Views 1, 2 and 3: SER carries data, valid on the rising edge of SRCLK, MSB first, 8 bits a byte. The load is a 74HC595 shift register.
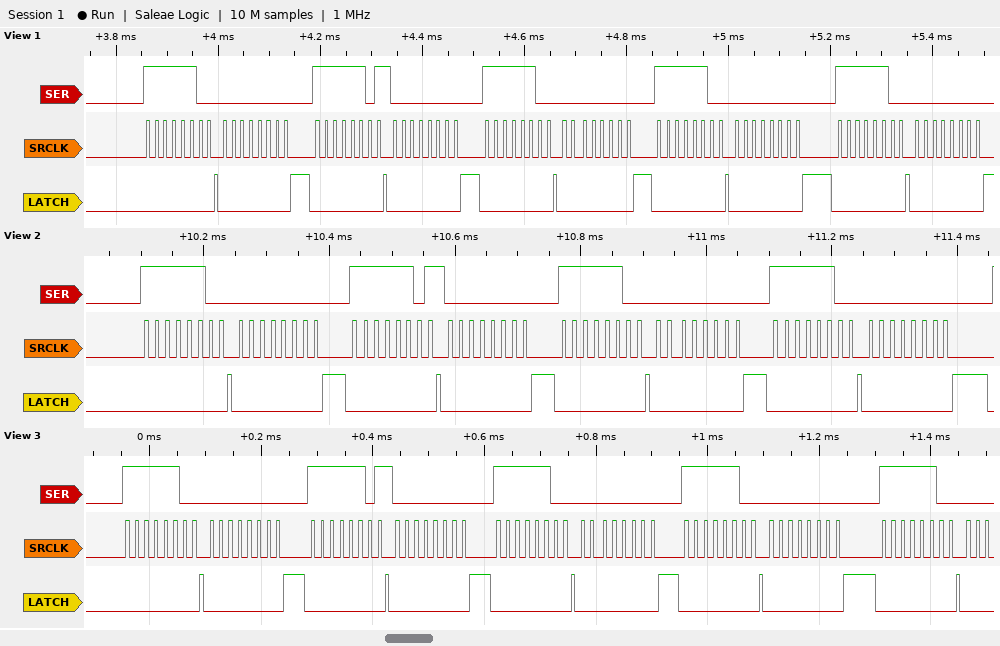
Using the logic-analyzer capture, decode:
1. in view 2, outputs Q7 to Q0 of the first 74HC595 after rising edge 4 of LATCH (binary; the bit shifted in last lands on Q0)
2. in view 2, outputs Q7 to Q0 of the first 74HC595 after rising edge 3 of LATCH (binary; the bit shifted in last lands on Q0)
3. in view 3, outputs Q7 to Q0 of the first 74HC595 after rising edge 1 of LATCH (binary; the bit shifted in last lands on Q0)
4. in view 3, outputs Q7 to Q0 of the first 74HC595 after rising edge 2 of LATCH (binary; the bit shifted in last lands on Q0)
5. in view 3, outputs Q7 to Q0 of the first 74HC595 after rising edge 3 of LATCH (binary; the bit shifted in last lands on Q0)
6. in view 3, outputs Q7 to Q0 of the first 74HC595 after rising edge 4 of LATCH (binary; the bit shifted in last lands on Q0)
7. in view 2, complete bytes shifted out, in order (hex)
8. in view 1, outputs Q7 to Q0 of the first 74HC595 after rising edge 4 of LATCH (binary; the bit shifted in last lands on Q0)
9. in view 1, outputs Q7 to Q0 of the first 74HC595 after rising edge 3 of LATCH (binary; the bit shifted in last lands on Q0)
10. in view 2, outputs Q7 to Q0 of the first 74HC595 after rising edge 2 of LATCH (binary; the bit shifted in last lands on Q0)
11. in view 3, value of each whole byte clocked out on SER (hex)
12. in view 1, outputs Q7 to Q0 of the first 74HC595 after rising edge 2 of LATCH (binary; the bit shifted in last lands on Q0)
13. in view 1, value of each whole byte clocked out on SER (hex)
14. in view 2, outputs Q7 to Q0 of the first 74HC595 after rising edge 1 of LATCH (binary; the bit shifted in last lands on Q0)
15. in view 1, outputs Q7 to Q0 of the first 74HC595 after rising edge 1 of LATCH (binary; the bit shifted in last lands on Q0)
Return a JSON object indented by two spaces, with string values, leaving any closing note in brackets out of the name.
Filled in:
{
  "in view 2, outputs Q7 to Q0 of the first 74HC595 after rising edge 4 of LATCH": "00000000",
  "in view 2, outputs Q7 to Q0 of the first 74HC595 after rising edge 3 of LATCH": "11111101",
  "in view 3, outputs Q7 to Q0 of the first 74HC595 after rising edge 1 of LATCH": "11111100",
  "in view 3, outputs Q7 to Q0 of the first 74HC595 after rising edge 2 of LATCH": "00000000",
  "in view 3, outputs Q7 to Q0 of the first 74HC595 after rising edge 3 of LATCH": "11111101",
  "in view 3, outputs Q7 to Q0 of the first 74HC595 after rising edge 4 of LATCH": "00000000",
  "in view 2, complete bytes shifted out, in order": "FC 00 FD 00 FC 00 FC 00",
  "in view 1, outputs Q7 to Q0 of the first 74HC595 after rising edge 4 of LATCH": "00000000",
  "in view 1, outputs Q7 to Q0 of the first 74HC595 after rising edge 3 of LATCH": "11111101",
  "in view 2, outputs Q7 to Q0 of the first 74HC595 after rising edge 2 of LATCH": "00000000",
  "in view 3, value of each whole byte clocked out on SER": "FC 00 FD 00 FC 00 FC 00 FC",
  "in view 1, outputs Q7 to Q0 of the first 74HC595 after rising edge 2 of LATCH": "00000000",
  "in view 1, value of each whole byte clocked out on SER": "0xFC 0x00 0xFD 0x00 0xFC 0x00 0xFC 0x00 0xFC 0x00",
  "in view 2, outputs Q7 to Q0 of the first 74HC595 after rising edge 1 of LATCH": "11111100",
  "in view 1, outputs Q7 to Q0 of the first 74HC595 after rising edge 1 of LATCH": "11111100"
}
